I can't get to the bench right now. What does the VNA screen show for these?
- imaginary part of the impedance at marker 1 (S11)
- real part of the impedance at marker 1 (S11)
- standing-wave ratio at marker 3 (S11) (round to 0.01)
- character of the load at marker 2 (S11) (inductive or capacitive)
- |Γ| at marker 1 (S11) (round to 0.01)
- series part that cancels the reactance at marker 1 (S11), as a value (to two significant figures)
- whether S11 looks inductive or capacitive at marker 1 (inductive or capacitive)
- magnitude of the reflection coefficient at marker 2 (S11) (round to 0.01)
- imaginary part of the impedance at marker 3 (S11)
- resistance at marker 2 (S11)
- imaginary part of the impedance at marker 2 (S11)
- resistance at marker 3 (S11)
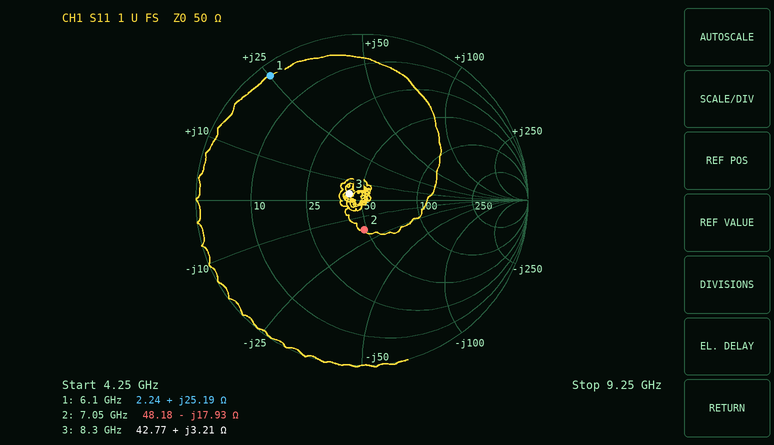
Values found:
+25.19 Ω
2.24 Ω
1.19
capacitive
0.93
1.0 pF
inductive
0.18
+3.21 Ω
48.18 Ω
-17.93 Ω
42.77 Ω
